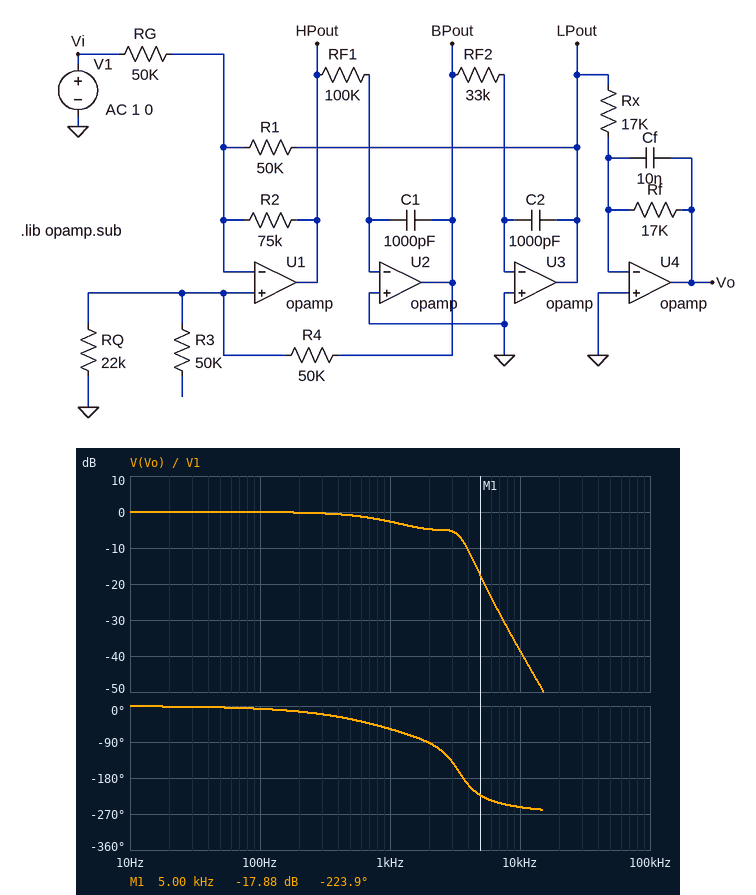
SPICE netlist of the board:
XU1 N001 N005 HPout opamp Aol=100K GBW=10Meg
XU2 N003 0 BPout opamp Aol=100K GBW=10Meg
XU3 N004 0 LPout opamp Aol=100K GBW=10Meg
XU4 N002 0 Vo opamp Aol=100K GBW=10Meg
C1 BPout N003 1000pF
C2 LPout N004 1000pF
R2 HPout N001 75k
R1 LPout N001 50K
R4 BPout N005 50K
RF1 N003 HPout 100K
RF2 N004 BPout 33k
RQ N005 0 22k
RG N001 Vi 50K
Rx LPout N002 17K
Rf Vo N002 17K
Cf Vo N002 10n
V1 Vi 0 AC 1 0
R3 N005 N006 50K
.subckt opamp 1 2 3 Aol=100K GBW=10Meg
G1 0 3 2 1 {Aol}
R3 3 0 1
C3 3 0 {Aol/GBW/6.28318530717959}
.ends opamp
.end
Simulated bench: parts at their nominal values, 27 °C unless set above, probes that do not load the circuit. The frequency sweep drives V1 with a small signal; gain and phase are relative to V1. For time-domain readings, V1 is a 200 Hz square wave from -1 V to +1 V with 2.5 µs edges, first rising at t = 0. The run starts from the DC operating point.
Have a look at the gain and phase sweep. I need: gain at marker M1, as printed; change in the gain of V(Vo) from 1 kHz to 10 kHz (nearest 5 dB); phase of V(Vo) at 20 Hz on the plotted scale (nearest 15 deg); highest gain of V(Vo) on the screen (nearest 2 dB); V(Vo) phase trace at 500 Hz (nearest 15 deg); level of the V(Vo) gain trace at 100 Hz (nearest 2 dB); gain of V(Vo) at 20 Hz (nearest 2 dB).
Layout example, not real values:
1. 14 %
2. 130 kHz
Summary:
1. -17.88 dB
2. -35 dB
3. 0 deg
4. 0 dB
5. -30 deg
6. 0 dB
7. 0 dB
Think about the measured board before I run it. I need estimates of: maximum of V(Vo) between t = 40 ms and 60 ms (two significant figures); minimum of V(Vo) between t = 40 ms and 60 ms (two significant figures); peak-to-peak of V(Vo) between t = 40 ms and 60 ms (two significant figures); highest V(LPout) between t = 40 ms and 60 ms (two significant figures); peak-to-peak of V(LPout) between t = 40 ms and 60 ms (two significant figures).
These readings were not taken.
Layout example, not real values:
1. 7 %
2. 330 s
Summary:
1. 1.0 V
2. -1.0 V
3. 2.0 V
4. 1.8 V
5. 3.6 V
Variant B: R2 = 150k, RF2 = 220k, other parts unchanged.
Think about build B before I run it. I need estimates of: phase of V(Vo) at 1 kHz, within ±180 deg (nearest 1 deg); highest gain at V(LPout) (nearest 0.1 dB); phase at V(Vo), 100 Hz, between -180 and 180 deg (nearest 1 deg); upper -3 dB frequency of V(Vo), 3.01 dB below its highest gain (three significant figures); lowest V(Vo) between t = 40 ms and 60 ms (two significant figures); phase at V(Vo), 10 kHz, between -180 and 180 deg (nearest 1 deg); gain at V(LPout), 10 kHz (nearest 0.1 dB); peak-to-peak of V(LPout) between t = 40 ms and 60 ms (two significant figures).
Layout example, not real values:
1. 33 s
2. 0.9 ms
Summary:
1. -101 deg
2. 0 dB
3. -12 deg
4. 736 Hz
5. -1.0 V
6. 114 deg
7. -29.4 dB
8. 2.0 V
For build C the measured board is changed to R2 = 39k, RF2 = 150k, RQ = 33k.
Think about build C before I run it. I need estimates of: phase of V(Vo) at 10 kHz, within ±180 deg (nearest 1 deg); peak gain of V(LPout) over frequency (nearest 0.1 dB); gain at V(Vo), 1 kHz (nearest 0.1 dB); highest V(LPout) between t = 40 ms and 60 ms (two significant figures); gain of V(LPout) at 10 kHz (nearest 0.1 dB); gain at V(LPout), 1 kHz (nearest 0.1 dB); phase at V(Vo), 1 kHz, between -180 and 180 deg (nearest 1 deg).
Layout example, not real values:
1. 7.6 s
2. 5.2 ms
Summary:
1. 104 deg
2. 0 dB
3. -5.3 dB
4. 1.1 V
5. -37.6 dB
6. -2.0 dB
7. -126 deg
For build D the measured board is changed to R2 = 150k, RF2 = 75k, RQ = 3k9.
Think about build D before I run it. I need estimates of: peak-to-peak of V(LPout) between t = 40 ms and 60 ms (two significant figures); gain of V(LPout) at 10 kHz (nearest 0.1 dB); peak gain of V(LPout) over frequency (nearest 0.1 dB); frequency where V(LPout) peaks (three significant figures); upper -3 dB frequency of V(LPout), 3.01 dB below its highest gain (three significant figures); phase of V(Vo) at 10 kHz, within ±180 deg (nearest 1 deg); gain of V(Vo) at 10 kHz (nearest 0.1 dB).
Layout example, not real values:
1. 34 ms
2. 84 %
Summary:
1. 4.7 V
2. -19.0 dB
3. 12.1 dB
4. 3.13 kHz
5. 3.51 kHz
6. 100 deg
7. -39.6 dB
